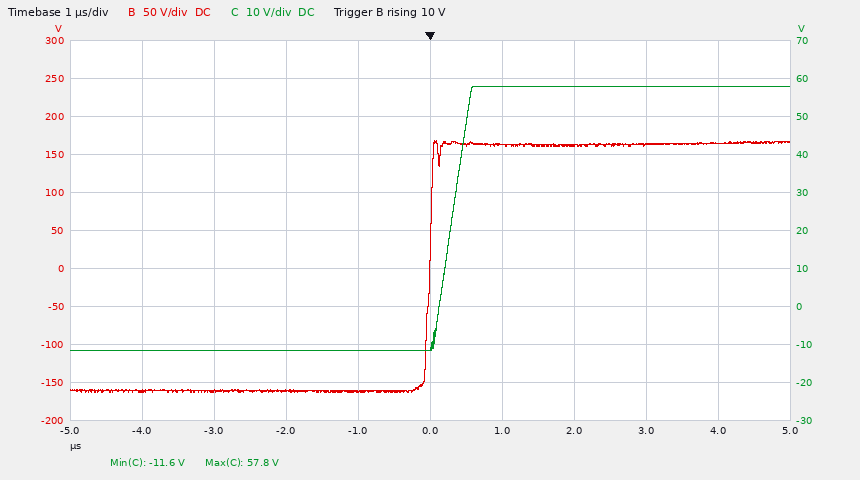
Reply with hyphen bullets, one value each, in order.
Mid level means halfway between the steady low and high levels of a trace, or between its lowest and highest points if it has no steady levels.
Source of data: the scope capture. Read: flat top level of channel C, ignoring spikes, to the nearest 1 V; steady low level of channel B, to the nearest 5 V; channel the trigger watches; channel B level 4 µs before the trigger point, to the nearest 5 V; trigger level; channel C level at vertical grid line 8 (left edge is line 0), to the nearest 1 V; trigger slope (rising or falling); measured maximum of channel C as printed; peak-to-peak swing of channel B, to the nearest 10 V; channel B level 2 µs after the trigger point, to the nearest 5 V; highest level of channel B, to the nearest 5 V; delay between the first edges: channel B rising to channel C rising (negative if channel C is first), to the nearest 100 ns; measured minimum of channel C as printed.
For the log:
- 58 V
- -160 V
- channel B
- -160 V
- 10 V
- 58 V
- rising
- 57.8 V
- 330 V
- 160 V
- 170 V
- +300 ns
- -11.6 V
